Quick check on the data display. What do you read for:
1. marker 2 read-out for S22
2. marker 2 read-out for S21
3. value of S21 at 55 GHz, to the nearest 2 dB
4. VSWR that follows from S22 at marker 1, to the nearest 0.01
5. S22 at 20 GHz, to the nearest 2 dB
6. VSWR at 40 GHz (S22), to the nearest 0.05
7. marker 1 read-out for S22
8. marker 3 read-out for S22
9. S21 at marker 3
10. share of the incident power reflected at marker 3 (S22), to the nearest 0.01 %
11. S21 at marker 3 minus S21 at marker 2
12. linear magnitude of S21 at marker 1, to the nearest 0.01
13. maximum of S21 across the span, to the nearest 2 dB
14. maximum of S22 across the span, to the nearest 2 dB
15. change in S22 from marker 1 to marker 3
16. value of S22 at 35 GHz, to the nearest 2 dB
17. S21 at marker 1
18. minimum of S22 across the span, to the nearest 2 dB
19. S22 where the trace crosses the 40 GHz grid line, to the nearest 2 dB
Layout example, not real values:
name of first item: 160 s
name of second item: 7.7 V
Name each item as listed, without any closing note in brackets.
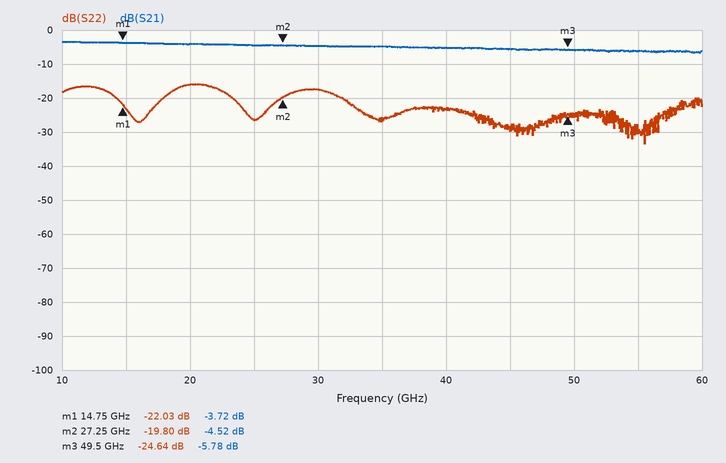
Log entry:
marker 2 read-out for S22: -19.80 dB
marker 2 read-out for S21: -4.52 dB
value of S21 at 55 GHz, to the nearest 2 dB: -6 dB
VSWR that follows from S22 at marker 1, to the nearest 0.01: 1.17
S22 at 20 GHz, to the nearest 2 dB: -16 dB
VSWR at 40 GHz (S22), to the nearest 0.05: 1.15
marker 1 read-out for S22: -22.03 dB
marker 3 read-out for S22: -24.64 dB
S21 at marker 3: -5.78 dB
share of the incident power reflected at marker 3 (S22), to the nearest 0.01 %: 0.34 %
S21 at marker 3 minus S21 at marker 2: -1.26 dB
linear magnitude of S21 at marker 1, to the nearest 0.01: 0.65
maximum of S21 across the span, to the nearest 2 dB: -4 dB
maximum of S22 across the span, to the nearest 2 dB: -16 dB
change in S22 from marker 1 to marker 3: -2.61 dB
value of S22 at 35 GHz, to the nearest 2 dB: -26 dB
S21 at marker 1: -3.72 dB
minimum of S22 across the span, to the nearest 2 dB: -34 dB
S22 where the trace crosses the 40 GHz grid line, to the nearest 2 dB: -24 dB
